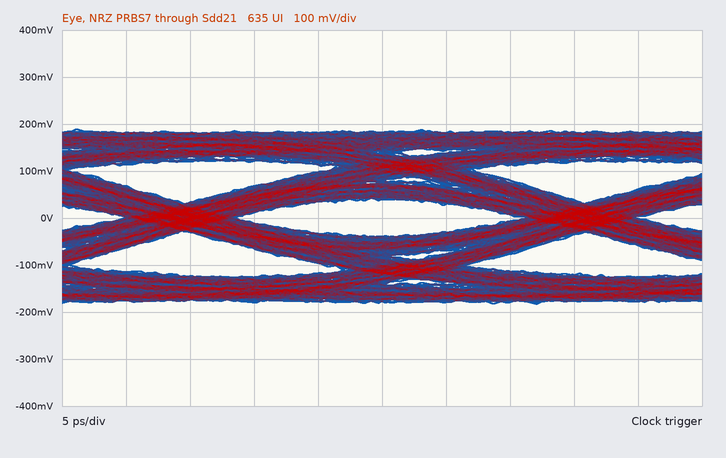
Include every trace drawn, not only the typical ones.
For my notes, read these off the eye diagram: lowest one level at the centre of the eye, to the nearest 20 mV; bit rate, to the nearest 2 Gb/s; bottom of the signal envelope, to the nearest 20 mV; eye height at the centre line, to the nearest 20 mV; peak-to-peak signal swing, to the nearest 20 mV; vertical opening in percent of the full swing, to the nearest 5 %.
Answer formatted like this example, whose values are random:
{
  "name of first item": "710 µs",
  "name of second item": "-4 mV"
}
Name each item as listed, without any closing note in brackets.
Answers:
{
  "lowest one level at the centre of the eye, to the nearest 20 mV": "40 mV",
  "bit rate, to the nearest 2 Gb/s": "32 Gb/s",
  "bottom of the signal envelope, to the nearest 20 mV": "-180 mV",
  "eye height at the centre line, to the nearest 20 mV": "80 mV",
  "peak-to-peak signal swing, to the nearest 20 mV": "380 mV",
  "vertical opening in percent of the full swing, to the nearest 5 %": "20 %"
}
